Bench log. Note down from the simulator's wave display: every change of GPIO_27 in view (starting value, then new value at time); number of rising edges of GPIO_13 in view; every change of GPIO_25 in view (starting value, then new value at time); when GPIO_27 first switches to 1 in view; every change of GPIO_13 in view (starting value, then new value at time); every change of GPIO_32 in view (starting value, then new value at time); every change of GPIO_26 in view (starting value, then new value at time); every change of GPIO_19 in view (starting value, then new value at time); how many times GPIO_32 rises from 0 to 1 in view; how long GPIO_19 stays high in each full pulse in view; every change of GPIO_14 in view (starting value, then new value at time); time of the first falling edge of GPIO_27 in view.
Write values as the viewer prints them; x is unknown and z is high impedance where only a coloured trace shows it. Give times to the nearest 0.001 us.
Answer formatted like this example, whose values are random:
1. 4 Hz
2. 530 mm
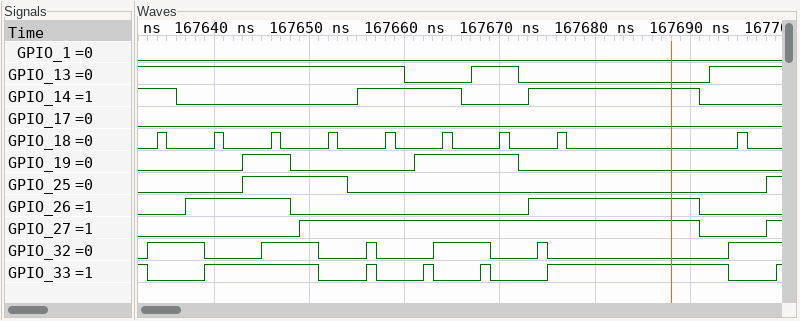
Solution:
1. 0, 1 at 167.649 us, 0 at 167.691 us, 1 at 167.698 us
2. 2
3. 0, 1 at 167.643 us, 0 at 167.654 us, 1 at 167.698 us
4. 167.649 us
5. 1, 0 at 167.66 us, 1 at 167.667 us, 0 at 167.672 us, 1 at 167.692 us
6. 0, 1 at 167.633 us, 0 at 167.639 us, 1 at 167.645 us, 0 at 167.651 us, 1 at 167.656 us, 0 at 167.657 us, 1 at 167.663 us, 0 at 167.669 us, 1 at 167.674 us, 0 at 167.675 us, 1 at 167.694 us
7. 0, 1 at 167.637 us, 0 at 167.648 us, 1 at 167.673 us, 0 at 167.691 us
8. 0, 1 at 167.643 us, 0 at 167.648 us, 1 at 167.661 us, 0 at 167.672 us
9. 6
10. 0.005 us, 0.011 us
11. 1, 0 at 167.636 us, 1 at 167.655 us, 0 at 167.666 us, 1 at 167.673 us, 0 at 167.691 us
12. 167.691 us
